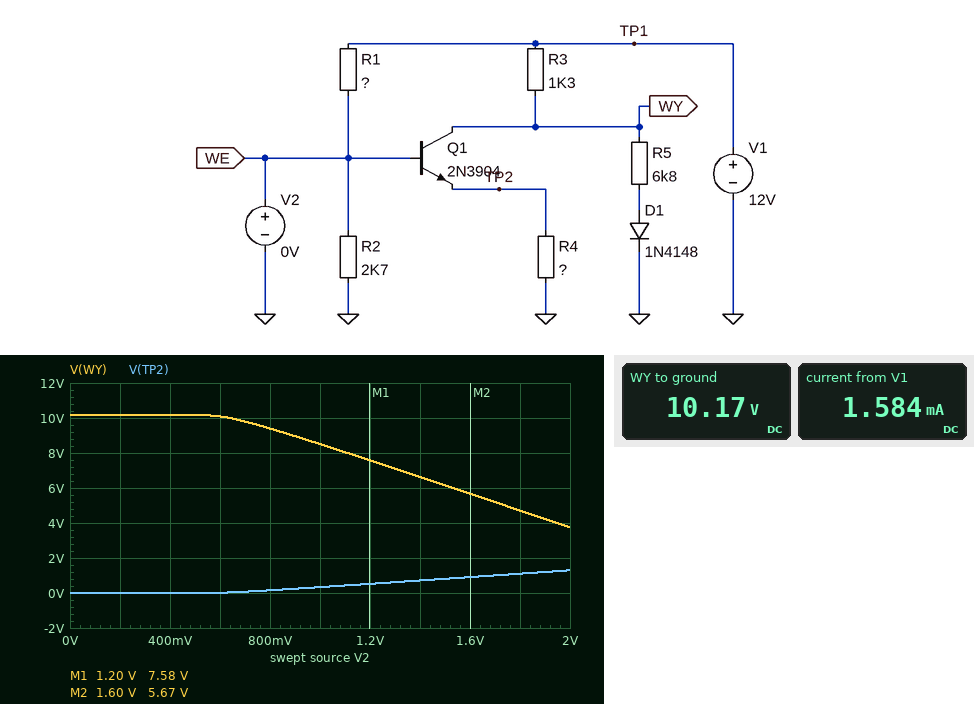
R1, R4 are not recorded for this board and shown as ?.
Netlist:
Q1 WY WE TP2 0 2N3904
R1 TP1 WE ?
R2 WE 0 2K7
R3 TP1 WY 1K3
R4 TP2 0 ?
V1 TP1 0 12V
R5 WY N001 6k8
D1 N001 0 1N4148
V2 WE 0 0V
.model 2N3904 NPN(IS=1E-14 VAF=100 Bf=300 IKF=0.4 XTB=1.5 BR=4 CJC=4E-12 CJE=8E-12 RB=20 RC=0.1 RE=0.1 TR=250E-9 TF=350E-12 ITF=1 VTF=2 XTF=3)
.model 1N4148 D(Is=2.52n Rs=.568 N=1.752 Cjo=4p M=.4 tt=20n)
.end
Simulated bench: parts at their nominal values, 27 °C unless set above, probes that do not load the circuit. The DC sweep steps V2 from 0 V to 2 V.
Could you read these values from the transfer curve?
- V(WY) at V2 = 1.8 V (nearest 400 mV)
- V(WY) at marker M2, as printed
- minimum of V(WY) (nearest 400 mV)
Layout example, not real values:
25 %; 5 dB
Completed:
4.8 V; 5.67 V; 3.6 V
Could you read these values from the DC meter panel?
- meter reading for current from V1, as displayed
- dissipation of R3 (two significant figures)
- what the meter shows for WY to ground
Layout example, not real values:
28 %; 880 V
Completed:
1.584 mA; 2.6 mW; 10.17 V
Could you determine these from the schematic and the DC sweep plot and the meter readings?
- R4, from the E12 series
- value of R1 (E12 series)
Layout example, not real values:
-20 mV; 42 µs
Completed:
220 Ω; 68 kΩ
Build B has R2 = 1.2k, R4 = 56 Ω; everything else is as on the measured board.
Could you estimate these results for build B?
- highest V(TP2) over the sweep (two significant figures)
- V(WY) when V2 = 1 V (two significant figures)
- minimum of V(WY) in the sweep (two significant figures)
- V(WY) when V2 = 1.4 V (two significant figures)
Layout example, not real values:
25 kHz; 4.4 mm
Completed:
1.0 V; 4.3 V; 570 mV; 640 mV
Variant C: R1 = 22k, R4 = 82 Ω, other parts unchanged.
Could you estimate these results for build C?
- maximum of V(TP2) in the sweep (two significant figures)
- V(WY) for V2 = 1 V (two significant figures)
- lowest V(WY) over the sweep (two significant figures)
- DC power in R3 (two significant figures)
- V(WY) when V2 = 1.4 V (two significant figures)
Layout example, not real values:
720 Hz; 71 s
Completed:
1.1 V; 6.0 V; 790 mV; 2.6 mW; 1.0 V
